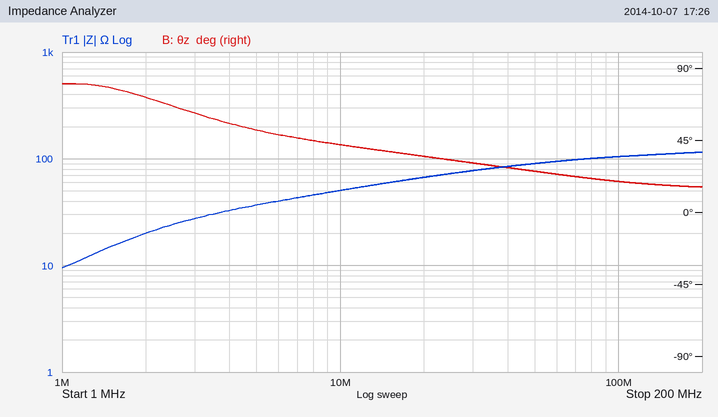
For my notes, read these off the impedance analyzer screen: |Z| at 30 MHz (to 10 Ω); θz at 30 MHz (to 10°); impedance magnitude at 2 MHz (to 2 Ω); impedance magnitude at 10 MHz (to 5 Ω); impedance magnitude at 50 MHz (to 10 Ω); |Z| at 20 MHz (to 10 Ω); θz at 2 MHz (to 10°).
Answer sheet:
80 Ω
30°
20 Ω
50 Ω
90 Ω
70 Ω
70°
